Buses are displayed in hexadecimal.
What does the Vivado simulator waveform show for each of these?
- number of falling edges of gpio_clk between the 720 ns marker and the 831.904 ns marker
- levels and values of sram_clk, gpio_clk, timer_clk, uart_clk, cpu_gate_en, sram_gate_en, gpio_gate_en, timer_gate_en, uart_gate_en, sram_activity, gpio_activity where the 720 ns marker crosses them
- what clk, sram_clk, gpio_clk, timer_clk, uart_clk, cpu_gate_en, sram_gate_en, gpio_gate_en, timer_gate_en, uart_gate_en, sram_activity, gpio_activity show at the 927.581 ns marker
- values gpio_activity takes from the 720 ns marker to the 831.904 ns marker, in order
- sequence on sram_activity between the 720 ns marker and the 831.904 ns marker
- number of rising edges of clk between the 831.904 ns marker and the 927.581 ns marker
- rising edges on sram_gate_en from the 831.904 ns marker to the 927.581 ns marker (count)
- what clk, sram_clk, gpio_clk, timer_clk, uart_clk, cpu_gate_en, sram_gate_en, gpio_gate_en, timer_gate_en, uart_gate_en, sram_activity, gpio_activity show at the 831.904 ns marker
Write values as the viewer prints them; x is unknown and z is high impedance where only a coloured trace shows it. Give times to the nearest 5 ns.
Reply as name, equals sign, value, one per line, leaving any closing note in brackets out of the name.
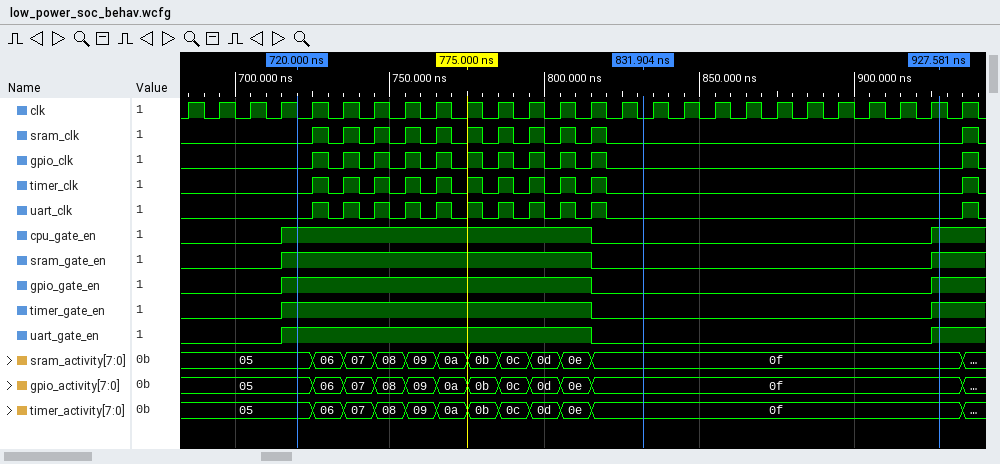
number of falling edges of gpio_clk between the 720 ns marker and the 831.904 ns marker = 10
levels and values of sram_clk, gpio_clk, timer_clk, uart_clk, cpu_gate_en, sram_gate_en, gpio_gate_en, timer_gate_en, uart_gate_en, sram_activity, gpio_activity where the 720 ns marker crosses them = sram_clk=0, gpio_clk=0, timer_clk=0, uart_clk=0, cpu_gate_en=1, sram_gate_en=1, gpio_gate_en=1, timer_gate_en=1, uart_gate_en=1, sram_activity=05, gpio_activity=05
what clk, sram_clk, gpio_clk, timer_clk, uart_clk, cpu_gate_en, sram_gate_en, gpio_gate_en, timer_gate_en, uart_gate_en, sram_activity, gpio_activity show at the 927.581 ns marker = clk=1, sram_clk=0, gpio_clk=0, timer_clk=0, uart_clk=0, cpu_gate_en=1, sram_gate_en=1, gpio_gate_en=1, timer_gate_en=1, uart_gate_en=1, sram_activity=0f, gpio_activity=0f
values gpio_activity takes from the 720 ns marker to the 831.904 ns marker, in order = 05, 06, 07, 08, 09, 0a, 0b, 0c, 0d, 0e, 0f
sequence on sram_activity between the 720 ns marker and the 831.904 ns marker = 05, 06, 07, 08, 09, 0a, 0b, 0c, 0d, 0e, 0f
number of rising edges of clk between the 831.904 ns marker and the 927.581 ns marker = 10
rising edges on sram_gate_en from the 831.904 ns marker to the 927.581 ns marker = 1
what clk, sram_clk, gpio_clk, timer_clk, uart_clk, cpu_gate_en, sram_gate_en, gpio_gate_en, timer_gate_en, uart_gate_en, sram_activity, gpio_activity show at the 831.904 ns marker = clk=0, sram_clk=0, gpio_clk=0, timer_clk=0, uart_clk=0, cpu_gate_en=0, sram_gate_en=0, gpio_gate_en=0, timer_gate_en=0, uart_gate_en=0, sram_activity=0f, gpio_activity=0f
